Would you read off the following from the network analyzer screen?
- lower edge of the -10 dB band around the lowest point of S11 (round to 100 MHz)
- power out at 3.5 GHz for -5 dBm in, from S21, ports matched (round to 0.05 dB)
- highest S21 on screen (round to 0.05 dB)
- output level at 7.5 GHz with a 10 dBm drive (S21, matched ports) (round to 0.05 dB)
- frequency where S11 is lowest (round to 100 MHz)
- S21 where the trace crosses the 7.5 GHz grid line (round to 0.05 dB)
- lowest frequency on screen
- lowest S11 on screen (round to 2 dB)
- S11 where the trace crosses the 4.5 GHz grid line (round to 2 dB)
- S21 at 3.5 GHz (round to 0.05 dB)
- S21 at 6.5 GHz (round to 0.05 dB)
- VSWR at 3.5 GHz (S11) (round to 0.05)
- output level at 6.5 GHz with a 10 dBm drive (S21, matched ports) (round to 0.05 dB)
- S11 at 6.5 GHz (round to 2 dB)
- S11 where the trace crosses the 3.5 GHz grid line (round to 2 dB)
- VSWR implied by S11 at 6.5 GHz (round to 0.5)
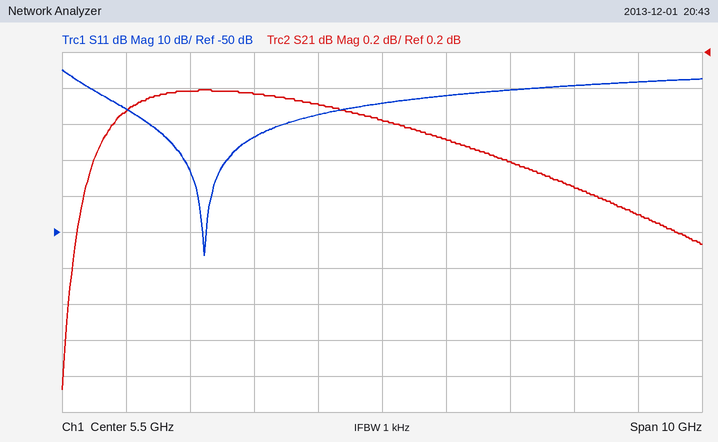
900 MHz
-5.05 dBm
0.00 dB
9.60 dBm
2.7 GHz
-0.40 dB
500 MHz
-56 dB
-18 dB
-0.05 dB
-0.30 dB
1.15
9.70 dBm
-12 dB
-24 dB
1.5
